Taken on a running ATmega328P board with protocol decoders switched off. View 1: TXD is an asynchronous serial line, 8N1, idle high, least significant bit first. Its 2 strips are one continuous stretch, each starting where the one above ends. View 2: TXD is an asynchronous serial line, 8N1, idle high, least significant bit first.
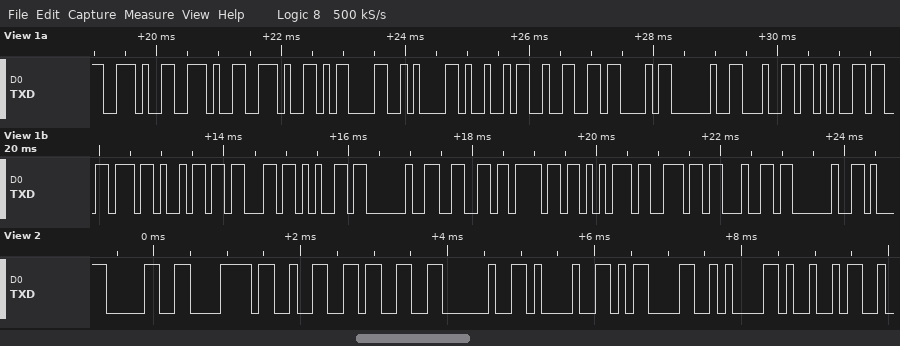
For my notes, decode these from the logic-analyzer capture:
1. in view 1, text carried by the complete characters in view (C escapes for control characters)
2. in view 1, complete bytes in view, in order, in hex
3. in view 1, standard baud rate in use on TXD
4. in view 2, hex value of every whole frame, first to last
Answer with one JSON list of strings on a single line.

["\"...\\r\\nI2C device found \"", "2E 2E 2E 0D 0A 49 32 43 20 64 65 76 69 63 65 20 66 6F 75 6E 64 20", "9600 baud", "30 78 32 33 20 21 0D 0A 49"]
